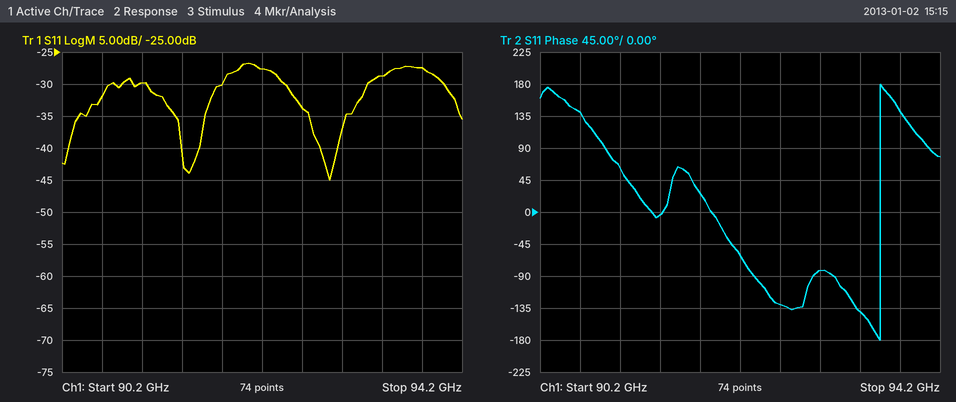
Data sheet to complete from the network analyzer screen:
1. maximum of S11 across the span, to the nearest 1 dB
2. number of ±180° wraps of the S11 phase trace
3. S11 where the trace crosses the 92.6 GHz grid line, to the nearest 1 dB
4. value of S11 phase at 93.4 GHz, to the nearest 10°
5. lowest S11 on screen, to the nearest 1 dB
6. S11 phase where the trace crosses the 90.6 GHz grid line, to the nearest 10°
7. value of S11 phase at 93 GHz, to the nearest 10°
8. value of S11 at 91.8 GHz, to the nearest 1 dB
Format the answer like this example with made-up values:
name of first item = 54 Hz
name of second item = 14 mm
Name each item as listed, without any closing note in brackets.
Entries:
maximum of S11 across the span, to the nearest 1 dB = -27 dB
number of ±180° wraps of the S11 phase trace = 1
S11 where the trace crosses the 92.6 GHz grid line, to the nearest 1 dB = -34 dB
value of S11 phase at 93.4 GHz, to the nearest 10° = -140°
lowest S11 on screen, to the nearest 1 dB = -45 dB
S11 phase where the trace crosses the 90.6 GHz grid line, to the nearest 10° = 140°
value of S11 phase at 93 GHz, to the nearest 10° = -80°
value of S11 at 91.8 GHz, to the nearest 1 dB = -30 dB
